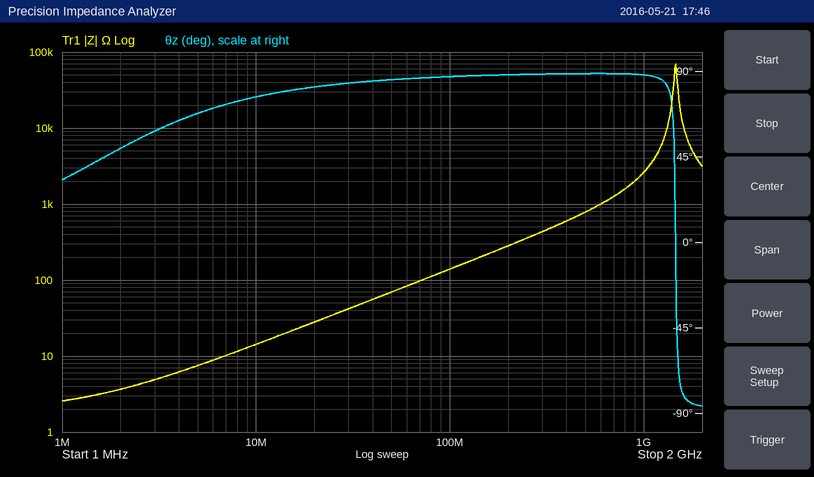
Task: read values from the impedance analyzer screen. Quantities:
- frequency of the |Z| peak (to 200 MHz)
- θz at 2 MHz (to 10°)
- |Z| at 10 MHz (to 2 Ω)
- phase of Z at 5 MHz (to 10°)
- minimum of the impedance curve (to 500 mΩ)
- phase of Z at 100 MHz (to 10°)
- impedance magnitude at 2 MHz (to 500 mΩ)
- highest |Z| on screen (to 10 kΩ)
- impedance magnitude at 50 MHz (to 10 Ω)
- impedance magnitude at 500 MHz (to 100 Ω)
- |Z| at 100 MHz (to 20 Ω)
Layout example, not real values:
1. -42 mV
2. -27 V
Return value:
1. 1.4 GHz
2. 50°
3. 14 Ω
4. 70°
5. 2.5 Ω
6. 90°
7. 3.5 Ω
8. 70 kΩ
9. 70 Ω
10. 800 Ω
11. 140 Ω
